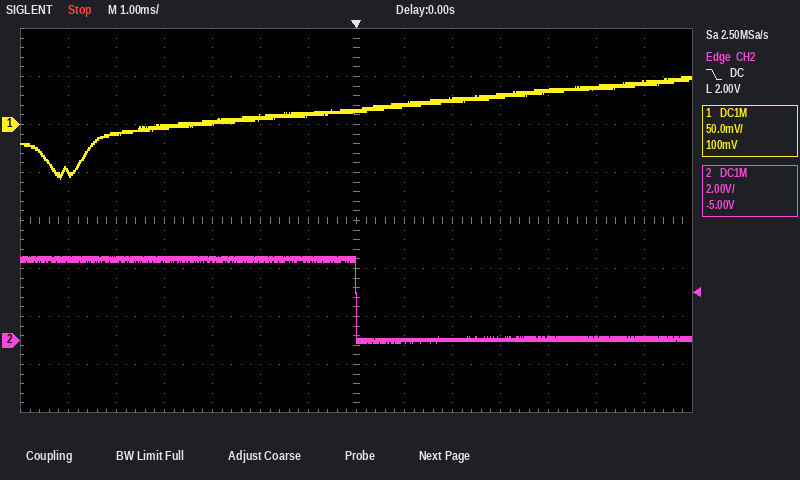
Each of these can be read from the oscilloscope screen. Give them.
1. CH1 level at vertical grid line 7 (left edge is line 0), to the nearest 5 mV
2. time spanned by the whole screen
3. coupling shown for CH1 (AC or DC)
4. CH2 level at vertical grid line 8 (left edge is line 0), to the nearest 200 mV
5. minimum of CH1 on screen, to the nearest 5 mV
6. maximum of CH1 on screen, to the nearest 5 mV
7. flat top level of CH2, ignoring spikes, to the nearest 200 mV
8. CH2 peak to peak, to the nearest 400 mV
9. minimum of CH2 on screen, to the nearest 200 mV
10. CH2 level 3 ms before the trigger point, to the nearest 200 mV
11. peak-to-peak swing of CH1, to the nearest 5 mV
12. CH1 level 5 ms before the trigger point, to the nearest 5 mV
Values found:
15 mV
14 ms
DC
0.0 V
-55 mV
50 mV
3.4 V
3.6 V
0.0 V
3.4 V
105 mV
-10 mV
